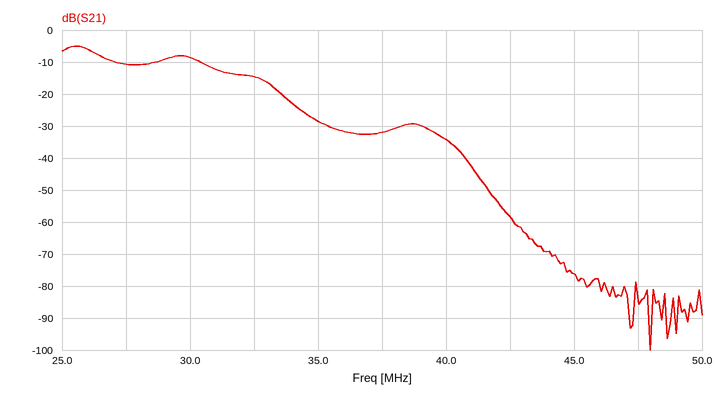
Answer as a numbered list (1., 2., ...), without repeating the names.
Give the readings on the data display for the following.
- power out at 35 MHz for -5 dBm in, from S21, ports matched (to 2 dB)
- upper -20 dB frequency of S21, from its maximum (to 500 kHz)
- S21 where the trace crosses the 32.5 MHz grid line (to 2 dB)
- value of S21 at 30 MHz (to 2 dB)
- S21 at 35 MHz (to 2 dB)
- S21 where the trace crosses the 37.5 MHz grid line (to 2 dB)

1. -34 dBm
2. 34.5 MHz
3. -14 dB
4. -8 dB
5. -28 dB
6. -32 dB
